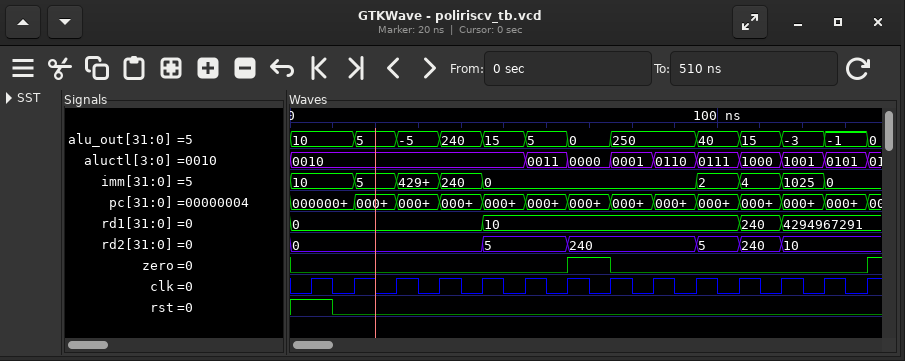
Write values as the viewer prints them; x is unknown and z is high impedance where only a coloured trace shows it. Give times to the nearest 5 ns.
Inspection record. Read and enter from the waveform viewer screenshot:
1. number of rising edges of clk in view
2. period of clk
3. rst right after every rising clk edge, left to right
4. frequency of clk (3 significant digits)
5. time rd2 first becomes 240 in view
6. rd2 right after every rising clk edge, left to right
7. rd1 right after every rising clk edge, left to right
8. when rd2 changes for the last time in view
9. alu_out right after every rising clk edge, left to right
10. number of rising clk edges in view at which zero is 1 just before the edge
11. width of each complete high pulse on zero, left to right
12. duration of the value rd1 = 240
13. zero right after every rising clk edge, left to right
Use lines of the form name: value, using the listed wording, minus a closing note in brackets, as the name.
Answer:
number of rising edges of clk in view: 14
period of clk: 10 ns
rst right after every rising clk edge, left to right: 1 0 0 0 0 0 0 0 0 0 0 0 0 0
frequency of clk: 100 MHz
time rd2 first becomes 240 in view: 65 ns
rd2 right after every rising clk edge, left to right: 0, 0, 0, 0, 5, 5, 240, 240, 240, 5, 240, 10, 10, 10
rd1 right after every rising clk edge, left to right: 0, 0, 0, 0, 10, 10, 10, 10, 10, 10, 240, 4294967291, 4294967291, 4294967291
when rd2 changes for the last time in view: 115 ns
alu_out right after every rising clk edge, left to right: 10, 5, -5, 240, 15, 5, 0, 250, 250, 40, 15, -3, -1, 0
number of rising clk edges in view at which zero is 1 just before the edge: 1
width of each complete high pulse on zero, left to right: 10 ns
duration of the value rd1 = 240: 10 ns
zero right after every rising clk edge, left to right: 0 0 0 0 0 0 1 0 0 0 0 0 0 1
